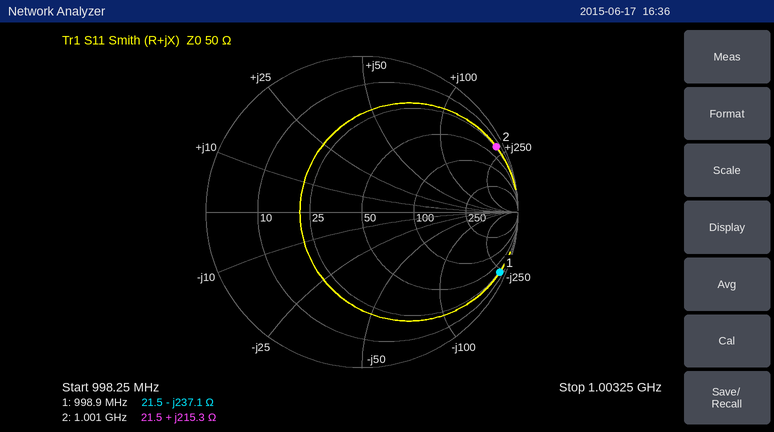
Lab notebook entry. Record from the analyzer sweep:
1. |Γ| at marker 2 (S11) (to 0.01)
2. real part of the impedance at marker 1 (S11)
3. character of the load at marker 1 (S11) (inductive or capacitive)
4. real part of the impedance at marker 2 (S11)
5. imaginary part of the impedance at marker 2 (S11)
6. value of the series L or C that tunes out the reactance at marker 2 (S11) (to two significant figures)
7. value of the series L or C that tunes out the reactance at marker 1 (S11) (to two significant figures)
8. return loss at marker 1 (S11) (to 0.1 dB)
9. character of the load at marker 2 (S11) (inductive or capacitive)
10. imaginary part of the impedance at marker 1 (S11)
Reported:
0.96
21.5 Ω
capacitive
21.5 Ω
+215.3 Ω
740 fF
38 nH
0.3 dB
inductive
-237.1 Ω
